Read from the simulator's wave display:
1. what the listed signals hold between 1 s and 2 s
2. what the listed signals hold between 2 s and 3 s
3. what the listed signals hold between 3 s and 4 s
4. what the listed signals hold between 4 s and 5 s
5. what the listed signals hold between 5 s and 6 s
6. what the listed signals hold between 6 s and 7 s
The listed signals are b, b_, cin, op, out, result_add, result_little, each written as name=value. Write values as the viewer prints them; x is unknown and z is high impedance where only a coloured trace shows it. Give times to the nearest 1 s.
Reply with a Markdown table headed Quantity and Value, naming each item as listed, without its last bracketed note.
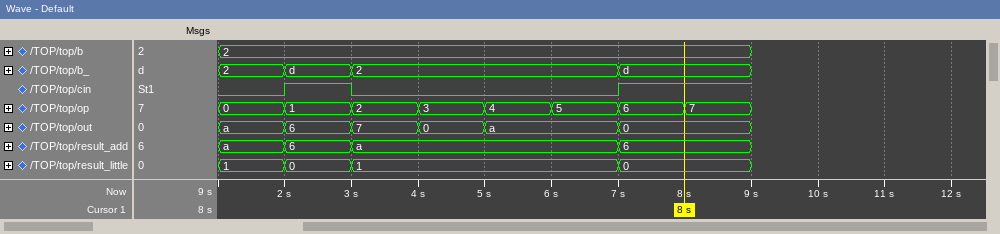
| Quantity | Value |
|---|---|
| what the listed signals hold between 1 s and 2 s | b=2, b_=2, cin=0, op=0, out=a, result_add=a, result_little=1 |
| what the listed signals hold between 2 s and 3 s | b=2, b_=d, cin=1, op=1, out=6, result_add=6, result_little=0 |
| what the listed signals hold between 3 s and 4 s | b=2, b_=2, cin=0, op=2, out=7, result_add=a, result_little=1 |
| what the listed signals hold between 4 s and 5 s | b=2, b_=2, cin=0, op=3, out=0, result_add=a, result_little=1 |
| what the listed signals hold between 5 s and 6 s | b=2, b_=2, cin=0, op=4, out=a, result_add=a, result_little=1 |
| what the listed signals hold between 6 s and 7 s | b=2, b_=2, cin=0, op=5, out=a, result_add=a, result_little=1 |
